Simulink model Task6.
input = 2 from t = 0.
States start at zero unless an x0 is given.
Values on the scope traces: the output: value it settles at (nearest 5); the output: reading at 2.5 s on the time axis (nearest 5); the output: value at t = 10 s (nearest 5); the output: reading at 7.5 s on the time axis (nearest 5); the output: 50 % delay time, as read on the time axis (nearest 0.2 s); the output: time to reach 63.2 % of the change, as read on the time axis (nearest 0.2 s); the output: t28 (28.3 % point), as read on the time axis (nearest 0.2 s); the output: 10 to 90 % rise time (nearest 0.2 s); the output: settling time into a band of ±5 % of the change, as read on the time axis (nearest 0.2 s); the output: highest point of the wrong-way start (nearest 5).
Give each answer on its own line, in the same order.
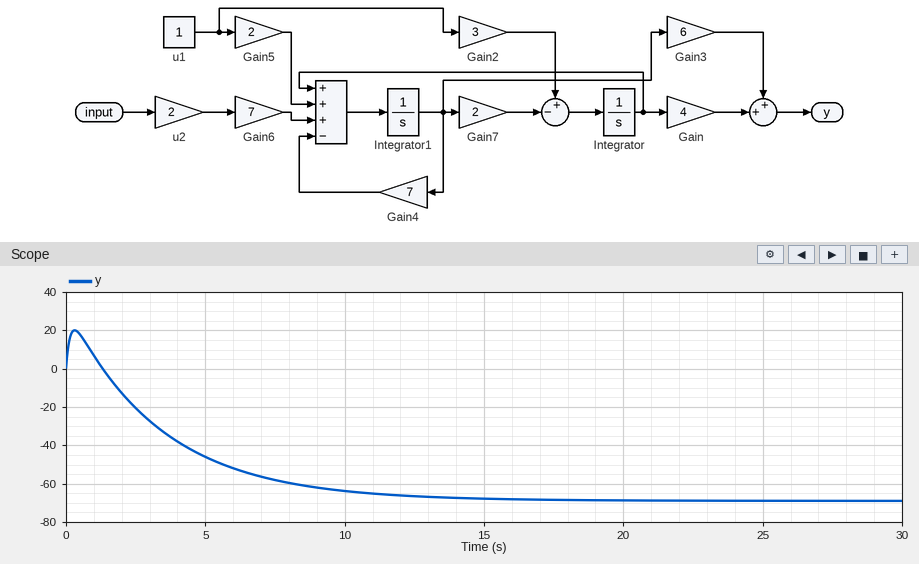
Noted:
-70
-20
-65
-60
3.6 s
4.6 s
2.4 s
7.4 s
11.4 s
20
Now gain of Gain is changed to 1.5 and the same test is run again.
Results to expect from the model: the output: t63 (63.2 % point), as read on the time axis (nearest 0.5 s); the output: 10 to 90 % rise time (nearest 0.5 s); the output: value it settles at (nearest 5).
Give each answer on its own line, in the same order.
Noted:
6.5 s
7.5 s
-20
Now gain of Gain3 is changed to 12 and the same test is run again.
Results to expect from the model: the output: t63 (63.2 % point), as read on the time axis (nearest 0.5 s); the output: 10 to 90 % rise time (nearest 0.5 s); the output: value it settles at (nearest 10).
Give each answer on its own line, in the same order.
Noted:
5.5 s
7.5 s
-60
